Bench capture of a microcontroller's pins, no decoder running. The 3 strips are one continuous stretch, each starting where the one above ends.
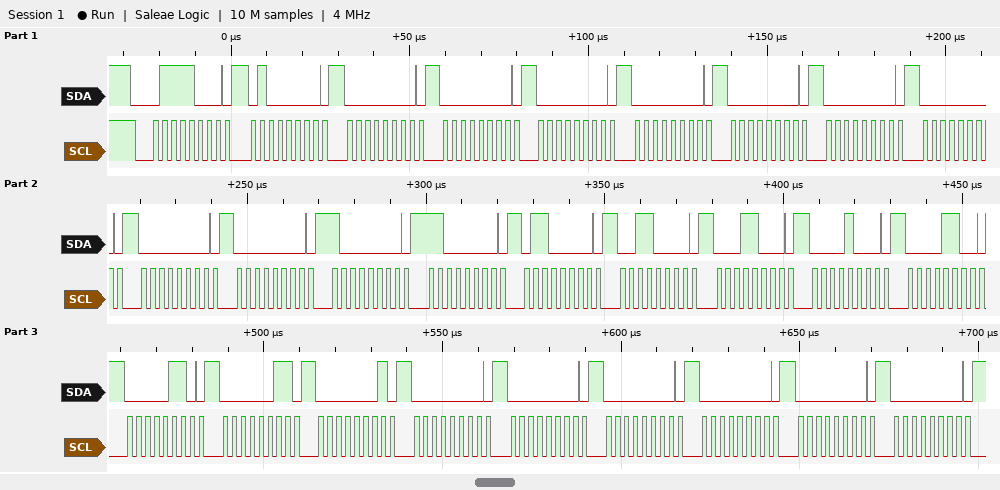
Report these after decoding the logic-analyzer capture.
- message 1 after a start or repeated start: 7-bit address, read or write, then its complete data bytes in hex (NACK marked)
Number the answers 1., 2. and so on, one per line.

1. 0x3C write: 40 00 00 00 00 00 00 00 00 00 80 C0 60 30 18 08 0C 06 03 01 00 00 00 00 00 00
